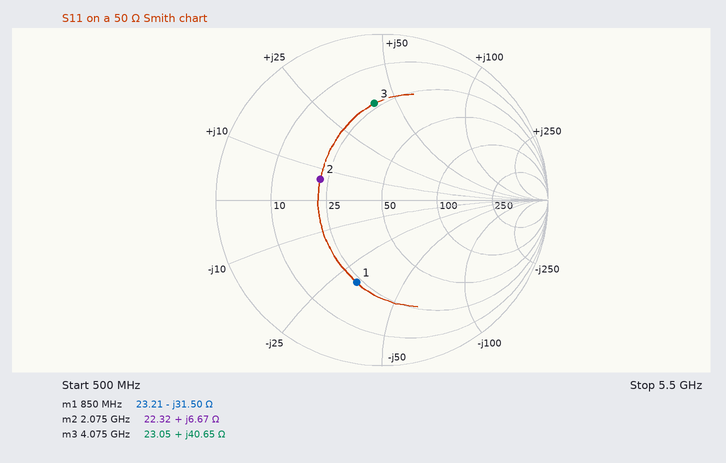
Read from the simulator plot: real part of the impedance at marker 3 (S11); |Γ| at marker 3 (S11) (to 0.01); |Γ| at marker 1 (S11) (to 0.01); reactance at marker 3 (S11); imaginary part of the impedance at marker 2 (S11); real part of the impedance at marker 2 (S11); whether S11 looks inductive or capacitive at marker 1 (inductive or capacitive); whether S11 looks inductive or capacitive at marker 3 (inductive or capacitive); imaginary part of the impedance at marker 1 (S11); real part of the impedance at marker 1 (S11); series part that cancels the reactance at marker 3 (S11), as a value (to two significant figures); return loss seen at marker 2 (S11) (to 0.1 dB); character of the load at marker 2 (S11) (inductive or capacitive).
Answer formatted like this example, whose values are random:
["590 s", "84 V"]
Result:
["23.05 Ω", "0.58", "0.52", "+40.65 Ω", "+6.67 Ω", "22.32 Ω", "capacitive", "inductive", "-31.50 Ω", "23.21 Ω", "960 fF", "8.1 dB", "inductive"]
